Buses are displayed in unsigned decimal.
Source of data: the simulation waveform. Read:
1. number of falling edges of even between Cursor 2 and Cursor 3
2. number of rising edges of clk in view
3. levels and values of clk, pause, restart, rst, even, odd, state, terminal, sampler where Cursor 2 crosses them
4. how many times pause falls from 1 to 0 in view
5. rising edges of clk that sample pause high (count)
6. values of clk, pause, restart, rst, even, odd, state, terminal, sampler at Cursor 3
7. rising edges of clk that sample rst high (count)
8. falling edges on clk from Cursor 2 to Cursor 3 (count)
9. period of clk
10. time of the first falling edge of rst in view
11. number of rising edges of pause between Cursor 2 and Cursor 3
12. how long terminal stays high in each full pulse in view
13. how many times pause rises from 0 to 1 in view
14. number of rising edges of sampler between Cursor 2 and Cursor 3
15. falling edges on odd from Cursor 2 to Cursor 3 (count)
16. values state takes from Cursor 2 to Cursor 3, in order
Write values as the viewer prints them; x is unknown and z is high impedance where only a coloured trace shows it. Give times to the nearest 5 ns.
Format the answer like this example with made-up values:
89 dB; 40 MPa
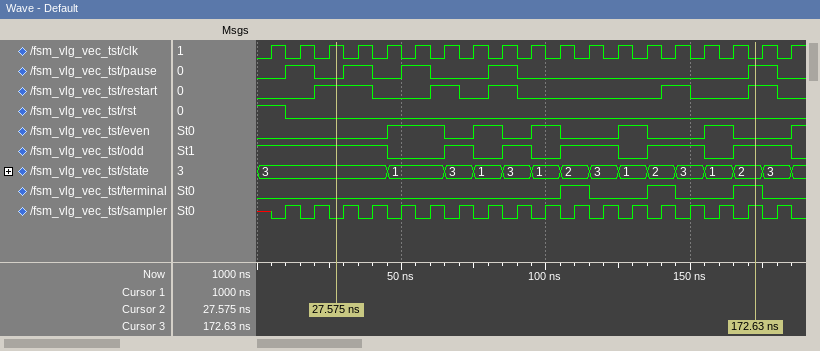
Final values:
5; 19; clk=1, pause=0, restart=1, rst=0, even=0, odd=1, state=3, terminal=0, sampler=0; 5; 5; clk=0, pause=1, restart=1, rst=0, even=0, odd=1, state=2, terminal=1, sampler=1; 1; 15; 10 ns; 10 ns; 4; 10 ns, 10 ns, 10 ns; 5; 15; 5; 3, 1, 3, 1, 3, 1, 2, 3, 1, 2, 3, 1, 2
